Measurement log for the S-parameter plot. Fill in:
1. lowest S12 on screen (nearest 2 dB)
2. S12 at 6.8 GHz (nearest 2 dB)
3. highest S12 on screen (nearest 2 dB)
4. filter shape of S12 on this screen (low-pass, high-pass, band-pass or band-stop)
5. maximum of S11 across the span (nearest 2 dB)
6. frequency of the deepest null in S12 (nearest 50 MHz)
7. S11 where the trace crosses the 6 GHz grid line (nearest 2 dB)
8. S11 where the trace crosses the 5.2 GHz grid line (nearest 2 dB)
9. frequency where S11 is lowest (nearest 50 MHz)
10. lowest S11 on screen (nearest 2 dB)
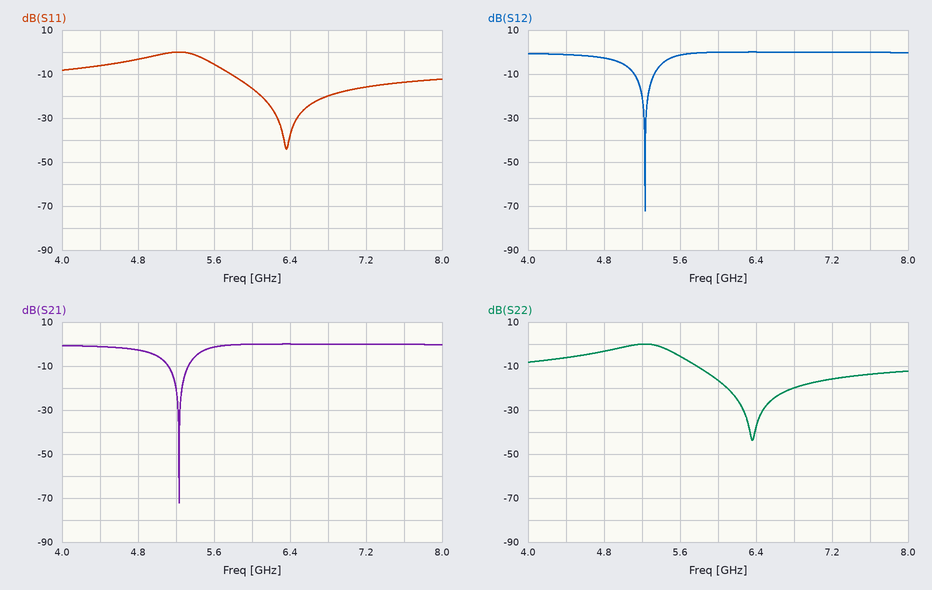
-72 dB
0 dB
0 dB
band-stop
0 dB
5.25 GHz
-16 dB
0 dB
6.35 GHz
-44 dB
